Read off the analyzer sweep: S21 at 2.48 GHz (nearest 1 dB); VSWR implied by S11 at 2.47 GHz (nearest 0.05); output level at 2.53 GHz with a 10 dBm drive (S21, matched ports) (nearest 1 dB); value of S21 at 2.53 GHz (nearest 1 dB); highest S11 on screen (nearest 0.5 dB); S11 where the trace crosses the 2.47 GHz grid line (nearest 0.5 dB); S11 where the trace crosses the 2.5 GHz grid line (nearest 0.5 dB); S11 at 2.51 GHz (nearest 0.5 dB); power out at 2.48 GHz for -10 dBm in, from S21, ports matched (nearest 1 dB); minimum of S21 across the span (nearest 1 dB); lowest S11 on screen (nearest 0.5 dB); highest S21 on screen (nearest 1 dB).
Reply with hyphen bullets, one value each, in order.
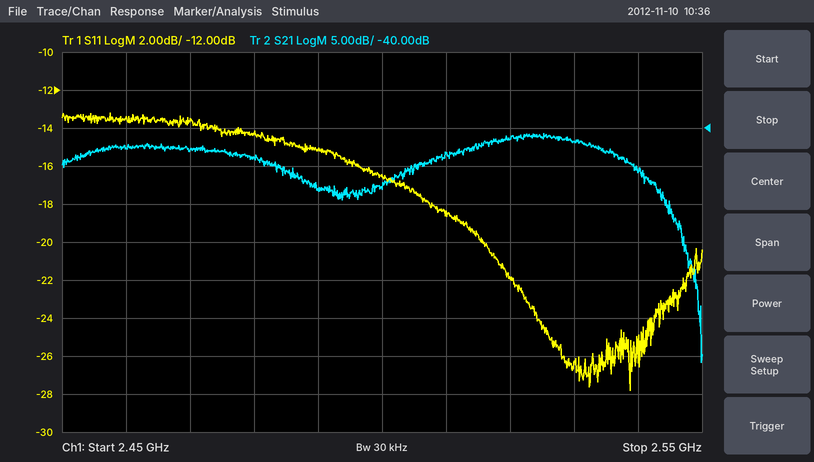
- -44 dB
- 1.55
- -32 dBm
- -42 dB
- -13.0 dB
- -13.5 dB
- -16.5 dB
- -18.5 dB
- -54 dBm
- -71 dB
- -28.0 dB
- -41 dB
